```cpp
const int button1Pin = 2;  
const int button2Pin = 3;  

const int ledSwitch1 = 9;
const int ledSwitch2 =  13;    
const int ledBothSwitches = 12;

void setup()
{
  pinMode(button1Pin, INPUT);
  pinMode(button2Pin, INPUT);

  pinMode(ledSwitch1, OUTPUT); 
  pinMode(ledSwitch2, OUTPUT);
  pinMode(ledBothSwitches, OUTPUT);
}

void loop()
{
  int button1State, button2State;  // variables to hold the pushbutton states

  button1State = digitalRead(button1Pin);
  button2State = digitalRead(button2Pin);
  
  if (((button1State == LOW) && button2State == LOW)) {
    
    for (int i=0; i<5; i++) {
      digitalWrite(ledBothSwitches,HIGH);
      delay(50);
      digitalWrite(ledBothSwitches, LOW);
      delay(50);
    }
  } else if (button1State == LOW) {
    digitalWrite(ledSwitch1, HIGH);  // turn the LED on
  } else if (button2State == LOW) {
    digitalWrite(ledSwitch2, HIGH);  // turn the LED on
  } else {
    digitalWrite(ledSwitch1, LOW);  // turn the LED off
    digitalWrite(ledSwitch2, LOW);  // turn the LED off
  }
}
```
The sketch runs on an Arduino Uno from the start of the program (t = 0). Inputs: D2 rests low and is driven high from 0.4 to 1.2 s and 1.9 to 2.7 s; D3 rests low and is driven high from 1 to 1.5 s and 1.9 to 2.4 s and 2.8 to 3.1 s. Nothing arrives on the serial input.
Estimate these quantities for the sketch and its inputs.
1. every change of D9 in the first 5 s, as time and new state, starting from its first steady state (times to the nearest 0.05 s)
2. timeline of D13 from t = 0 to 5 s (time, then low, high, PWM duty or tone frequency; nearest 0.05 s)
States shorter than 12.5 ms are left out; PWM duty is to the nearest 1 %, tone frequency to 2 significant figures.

0 s low; 1.2 s high; 2 s low
0 s low; 0.5 s high; 1 s low; 2.4 s high
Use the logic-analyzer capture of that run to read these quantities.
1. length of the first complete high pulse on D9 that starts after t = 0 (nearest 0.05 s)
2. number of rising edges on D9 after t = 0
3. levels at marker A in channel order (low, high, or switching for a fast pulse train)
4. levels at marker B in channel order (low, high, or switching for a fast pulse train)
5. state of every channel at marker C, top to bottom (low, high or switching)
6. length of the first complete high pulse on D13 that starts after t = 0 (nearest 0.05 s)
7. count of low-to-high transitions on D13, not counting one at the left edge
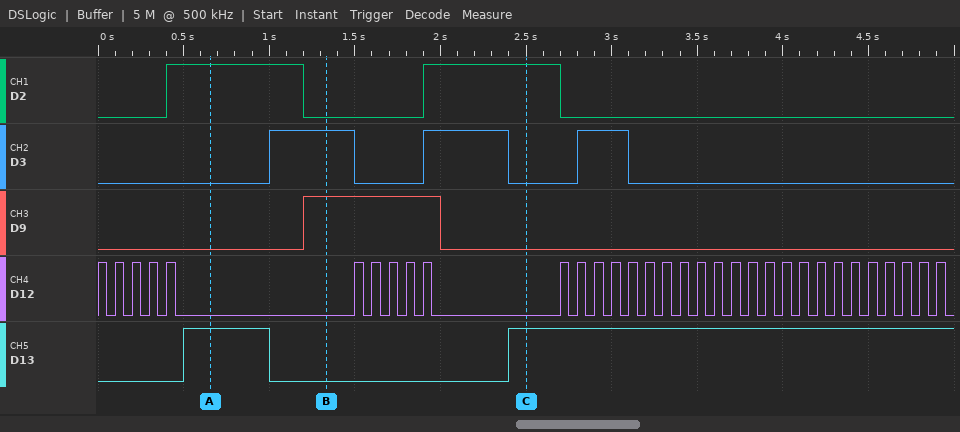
0.80 s
1
D2 high, D3 low, D9 low, D12 low, D13 high
D2 low, D3 high, D9 high, D12 low, D13 low
D2 high, D3 low, D9 low, D12 low, D13 high
0.50 s
2
